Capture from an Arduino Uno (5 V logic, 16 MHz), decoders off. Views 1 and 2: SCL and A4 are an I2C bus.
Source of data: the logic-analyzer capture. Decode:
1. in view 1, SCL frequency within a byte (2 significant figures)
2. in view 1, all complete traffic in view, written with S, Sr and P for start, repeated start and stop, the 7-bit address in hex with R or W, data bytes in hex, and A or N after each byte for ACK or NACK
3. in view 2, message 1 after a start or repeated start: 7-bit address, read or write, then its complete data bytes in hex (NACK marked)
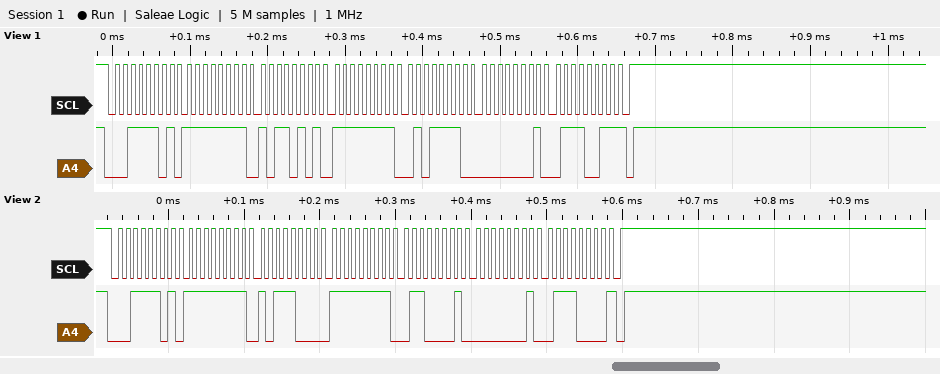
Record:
100 kHz
S 1ER A FF A B5 A FF A 5E A 01 A 73 N P
0x1E read: FF B8 FF 61 01 70 NACK
